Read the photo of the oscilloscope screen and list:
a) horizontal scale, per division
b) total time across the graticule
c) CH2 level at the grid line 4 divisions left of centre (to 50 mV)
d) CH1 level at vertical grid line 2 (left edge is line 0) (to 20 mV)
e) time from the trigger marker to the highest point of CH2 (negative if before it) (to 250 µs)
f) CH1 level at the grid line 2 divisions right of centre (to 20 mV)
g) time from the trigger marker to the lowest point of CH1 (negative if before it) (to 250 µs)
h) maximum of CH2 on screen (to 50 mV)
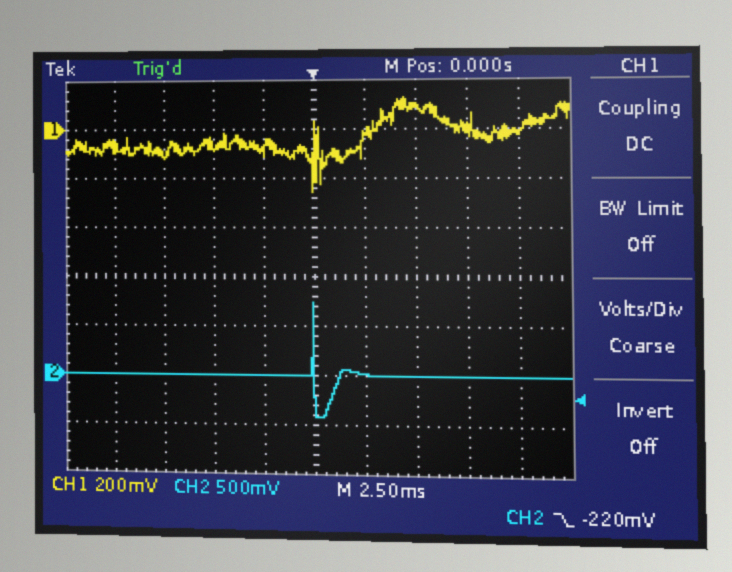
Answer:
2.5 ms
25 ms
0 mV
-100 mV
0.00 ms
100 mV
0.00 ms
750 mV
